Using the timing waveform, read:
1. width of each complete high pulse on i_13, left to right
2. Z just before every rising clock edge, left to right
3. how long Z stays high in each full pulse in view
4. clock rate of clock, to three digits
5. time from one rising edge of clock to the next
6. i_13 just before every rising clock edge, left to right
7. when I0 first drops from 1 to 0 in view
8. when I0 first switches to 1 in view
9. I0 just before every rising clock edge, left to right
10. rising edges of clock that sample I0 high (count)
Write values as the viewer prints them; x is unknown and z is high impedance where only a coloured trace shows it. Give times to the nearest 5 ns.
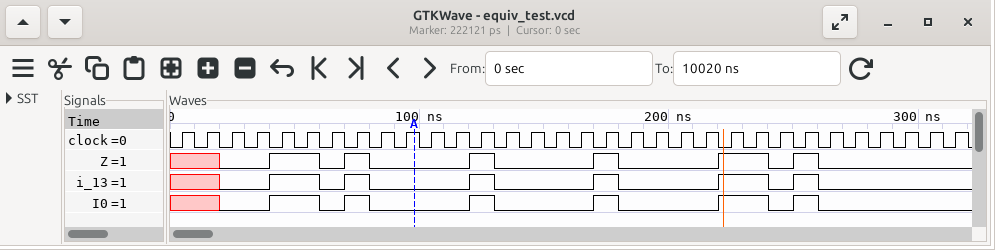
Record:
20 ns, 10 ns, 10 ns, 10 ns, 20 ns, 10 ns
x x 0 0 1 1 0 1 0 0 0 0 1 0 0 0 0 1 0 0 0 0 1 1 0 1 0 0 0 0 0 0
20 ns, 10 ns, 10 ns, 10 ns, 20 ns, 10 ns
100 MHz
10 ns
x x 0 0 1 1 0 1 0 0 0 0 1 0 0 0 0 1 0 0 0 0 1 1 0 1 0 0 0 0 0 0
60 ns
40 ns
x x 0 0 1 1 0 1 0 0 0 0 1 0 0 0 0 1 0 0 0 0 1 1 0 1 0 0 0 0 0 0
8
